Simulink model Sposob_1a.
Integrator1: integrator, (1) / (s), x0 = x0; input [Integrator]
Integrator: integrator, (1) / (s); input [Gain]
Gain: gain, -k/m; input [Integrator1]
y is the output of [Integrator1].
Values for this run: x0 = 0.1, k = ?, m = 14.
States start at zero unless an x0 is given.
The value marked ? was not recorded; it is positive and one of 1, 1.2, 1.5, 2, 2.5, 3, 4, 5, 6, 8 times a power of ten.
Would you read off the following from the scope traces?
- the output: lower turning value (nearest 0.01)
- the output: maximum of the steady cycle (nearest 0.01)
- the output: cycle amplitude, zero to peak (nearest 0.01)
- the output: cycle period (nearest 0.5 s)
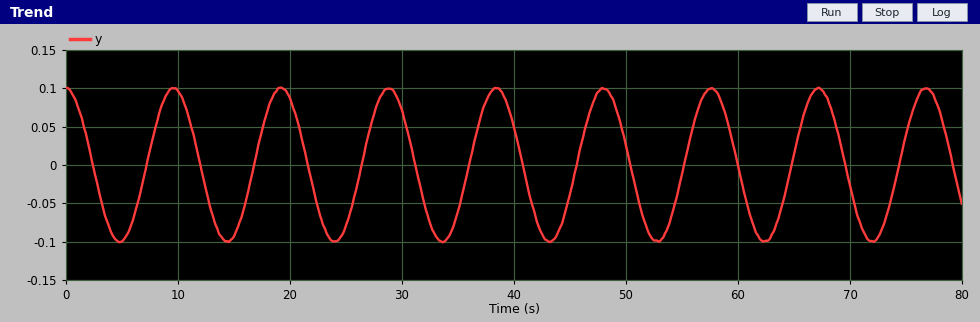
-0.10
0.10
0.10
9.5 s
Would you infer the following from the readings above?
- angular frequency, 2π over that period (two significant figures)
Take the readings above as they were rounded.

0.66 rad/s
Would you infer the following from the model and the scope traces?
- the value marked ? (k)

6
